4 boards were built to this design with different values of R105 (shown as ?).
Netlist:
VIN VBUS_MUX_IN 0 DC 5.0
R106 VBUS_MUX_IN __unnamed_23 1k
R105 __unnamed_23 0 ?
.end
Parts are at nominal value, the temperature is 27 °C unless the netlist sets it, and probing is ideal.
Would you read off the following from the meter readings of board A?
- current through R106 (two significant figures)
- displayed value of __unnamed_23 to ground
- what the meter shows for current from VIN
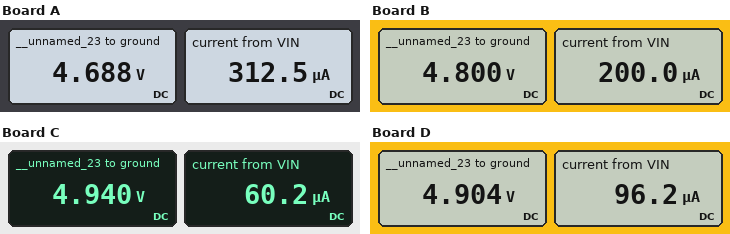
310 µA
4.688 V
312.5 µA
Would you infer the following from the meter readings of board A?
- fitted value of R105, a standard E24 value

15 kΩ
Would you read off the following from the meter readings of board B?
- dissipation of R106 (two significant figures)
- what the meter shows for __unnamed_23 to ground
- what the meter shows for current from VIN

40 µW
4.800 V
200.0 µA
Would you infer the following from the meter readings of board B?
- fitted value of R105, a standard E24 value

24 kΩ
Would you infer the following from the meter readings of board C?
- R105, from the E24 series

82 kΩ
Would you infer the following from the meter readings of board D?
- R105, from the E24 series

51 kΩ
